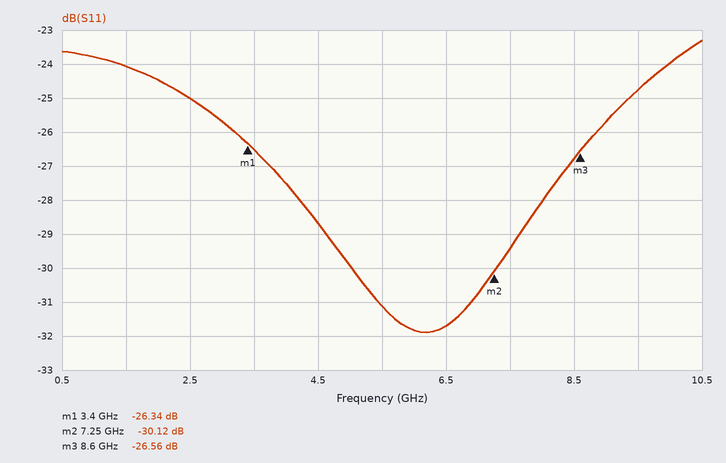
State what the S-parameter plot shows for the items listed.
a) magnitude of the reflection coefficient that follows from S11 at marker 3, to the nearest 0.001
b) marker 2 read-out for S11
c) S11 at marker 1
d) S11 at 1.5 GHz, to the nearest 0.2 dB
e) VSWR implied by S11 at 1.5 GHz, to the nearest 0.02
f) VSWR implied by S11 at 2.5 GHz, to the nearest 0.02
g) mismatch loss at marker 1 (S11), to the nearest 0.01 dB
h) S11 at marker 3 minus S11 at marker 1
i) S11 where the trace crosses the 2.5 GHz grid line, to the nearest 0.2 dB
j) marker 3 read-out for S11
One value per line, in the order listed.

0.047
-30.12 dB
-26.34 dB
-24.0 dB
1.14
1.12
0.01 dB
-0.22 dB
-25.0 dB
-26.56 dB
